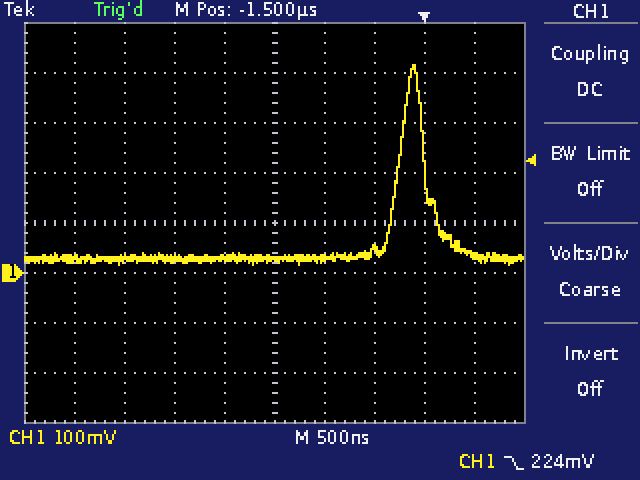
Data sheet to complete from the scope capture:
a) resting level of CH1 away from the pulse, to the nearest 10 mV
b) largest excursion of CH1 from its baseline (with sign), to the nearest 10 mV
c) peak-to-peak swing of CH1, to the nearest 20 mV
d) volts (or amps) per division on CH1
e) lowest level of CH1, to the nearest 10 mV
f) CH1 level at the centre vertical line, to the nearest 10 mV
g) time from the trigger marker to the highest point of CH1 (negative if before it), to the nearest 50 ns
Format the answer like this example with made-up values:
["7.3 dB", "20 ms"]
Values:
["30 mV", "+390 mV", "400 mV", "100 mV", "20 mV", "30 mV", "-100 ns"]
